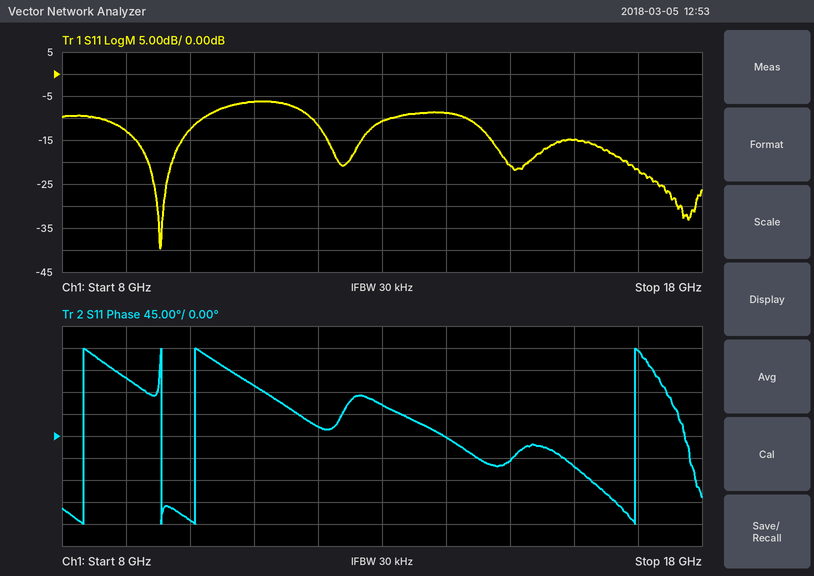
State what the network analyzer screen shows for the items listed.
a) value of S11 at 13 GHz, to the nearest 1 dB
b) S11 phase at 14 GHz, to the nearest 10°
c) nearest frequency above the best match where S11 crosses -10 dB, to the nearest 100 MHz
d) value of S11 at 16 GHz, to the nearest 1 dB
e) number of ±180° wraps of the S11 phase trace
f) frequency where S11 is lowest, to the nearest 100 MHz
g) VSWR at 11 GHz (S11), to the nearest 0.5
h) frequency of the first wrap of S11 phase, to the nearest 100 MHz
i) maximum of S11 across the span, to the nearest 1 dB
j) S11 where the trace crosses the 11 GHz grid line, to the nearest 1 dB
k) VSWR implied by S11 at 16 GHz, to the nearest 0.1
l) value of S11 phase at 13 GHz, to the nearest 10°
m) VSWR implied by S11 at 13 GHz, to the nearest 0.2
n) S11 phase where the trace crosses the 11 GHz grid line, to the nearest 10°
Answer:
-11 dB
0°
10.2 GHz
-15 dB
4
9.5 GHz
3.0
8.3 GHz
-6 dB
-6 dB
1.4
60°
1.8
100°
